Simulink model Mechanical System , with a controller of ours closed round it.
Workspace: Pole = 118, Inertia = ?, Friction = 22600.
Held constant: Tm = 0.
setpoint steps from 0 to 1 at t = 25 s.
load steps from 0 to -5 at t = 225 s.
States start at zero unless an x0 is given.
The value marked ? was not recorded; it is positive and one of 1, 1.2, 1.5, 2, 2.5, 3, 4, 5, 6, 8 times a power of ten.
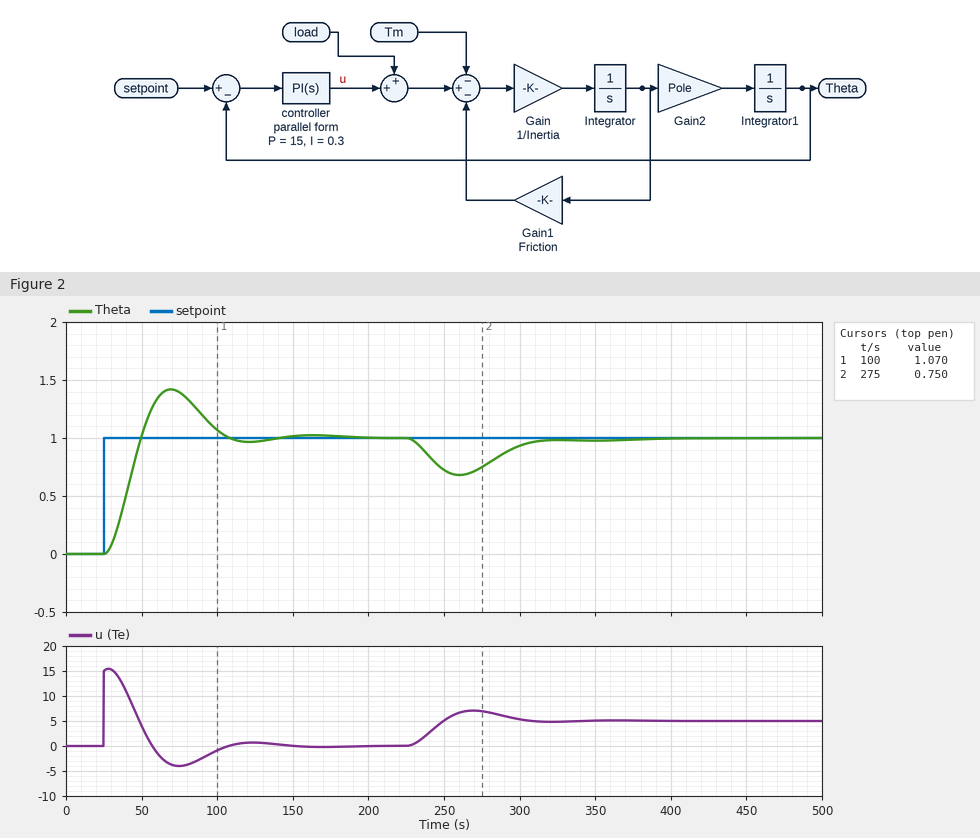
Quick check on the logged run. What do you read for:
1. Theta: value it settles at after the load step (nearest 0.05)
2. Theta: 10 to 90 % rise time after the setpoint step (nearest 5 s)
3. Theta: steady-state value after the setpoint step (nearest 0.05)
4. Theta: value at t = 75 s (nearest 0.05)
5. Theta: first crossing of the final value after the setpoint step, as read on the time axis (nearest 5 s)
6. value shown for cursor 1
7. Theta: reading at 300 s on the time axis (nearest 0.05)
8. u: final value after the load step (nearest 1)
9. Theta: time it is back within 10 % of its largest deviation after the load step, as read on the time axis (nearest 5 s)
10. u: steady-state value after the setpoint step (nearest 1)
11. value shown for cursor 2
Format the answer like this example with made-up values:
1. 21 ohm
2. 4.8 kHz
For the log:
1. 1.00
2. 15 s
3. 1.00
4. 1.40
5. 50 s
6. 1.070
7. 0.95
8. 5
9. 310 s
10. 0
11. 0.750
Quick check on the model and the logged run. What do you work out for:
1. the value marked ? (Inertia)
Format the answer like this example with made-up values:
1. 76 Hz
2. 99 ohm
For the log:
1. 250000
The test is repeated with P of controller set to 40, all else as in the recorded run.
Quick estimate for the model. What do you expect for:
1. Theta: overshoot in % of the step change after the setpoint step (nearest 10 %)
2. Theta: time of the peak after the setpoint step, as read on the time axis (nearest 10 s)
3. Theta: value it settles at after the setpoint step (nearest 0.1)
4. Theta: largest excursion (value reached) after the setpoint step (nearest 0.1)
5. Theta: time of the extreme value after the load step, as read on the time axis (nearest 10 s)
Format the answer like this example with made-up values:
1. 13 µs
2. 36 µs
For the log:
1. 40 %
2. 50 s
3. 1.0
4. 1.4
5. 250 s
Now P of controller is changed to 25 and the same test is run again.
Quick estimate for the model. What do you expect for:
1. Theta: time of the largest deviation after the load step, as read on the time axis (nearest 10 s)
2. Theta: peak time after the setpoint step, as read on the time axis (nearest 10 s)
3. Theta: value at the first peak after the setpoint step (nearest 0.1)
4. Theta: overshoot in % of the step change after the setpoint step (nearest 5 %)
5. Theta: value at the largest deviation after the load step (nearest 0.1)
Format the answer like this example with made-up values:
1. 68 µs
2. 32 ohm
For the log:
1. 250 s
2. 60 s
3. 1.4
4. 40 %
5. 0.8
